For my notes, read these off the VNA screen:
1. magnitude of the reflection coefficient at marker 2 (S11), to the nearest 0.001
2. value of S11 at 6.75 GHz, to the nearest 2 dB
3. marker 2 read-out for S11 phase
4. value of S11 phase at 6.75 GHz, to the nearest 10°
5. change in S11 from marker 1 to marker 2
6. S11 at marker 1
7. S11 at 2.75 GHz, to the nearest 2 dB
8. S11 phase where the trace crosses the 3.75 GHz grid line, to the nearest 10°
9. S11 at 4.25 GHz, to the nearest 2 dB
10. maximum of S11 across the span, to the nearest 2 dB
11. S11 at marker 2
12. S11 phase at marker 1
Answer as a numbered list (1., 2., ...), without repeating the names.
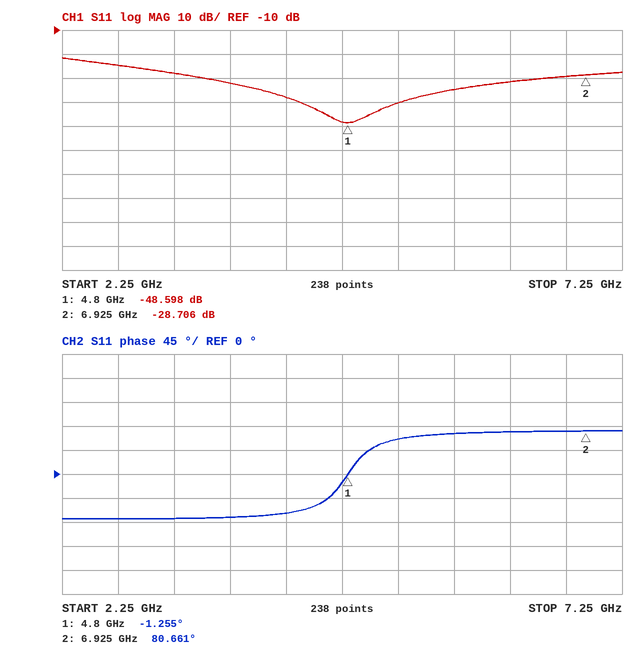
1. 0.037
2. -30 dB
3. 80.661°
4. 80°
5. 19.892 dB
6. -48.598 dB
7. -24 dB
8. -80°
9. -38 dB
10. -22 dB
11. -28.706 dB
12. -1.255°
